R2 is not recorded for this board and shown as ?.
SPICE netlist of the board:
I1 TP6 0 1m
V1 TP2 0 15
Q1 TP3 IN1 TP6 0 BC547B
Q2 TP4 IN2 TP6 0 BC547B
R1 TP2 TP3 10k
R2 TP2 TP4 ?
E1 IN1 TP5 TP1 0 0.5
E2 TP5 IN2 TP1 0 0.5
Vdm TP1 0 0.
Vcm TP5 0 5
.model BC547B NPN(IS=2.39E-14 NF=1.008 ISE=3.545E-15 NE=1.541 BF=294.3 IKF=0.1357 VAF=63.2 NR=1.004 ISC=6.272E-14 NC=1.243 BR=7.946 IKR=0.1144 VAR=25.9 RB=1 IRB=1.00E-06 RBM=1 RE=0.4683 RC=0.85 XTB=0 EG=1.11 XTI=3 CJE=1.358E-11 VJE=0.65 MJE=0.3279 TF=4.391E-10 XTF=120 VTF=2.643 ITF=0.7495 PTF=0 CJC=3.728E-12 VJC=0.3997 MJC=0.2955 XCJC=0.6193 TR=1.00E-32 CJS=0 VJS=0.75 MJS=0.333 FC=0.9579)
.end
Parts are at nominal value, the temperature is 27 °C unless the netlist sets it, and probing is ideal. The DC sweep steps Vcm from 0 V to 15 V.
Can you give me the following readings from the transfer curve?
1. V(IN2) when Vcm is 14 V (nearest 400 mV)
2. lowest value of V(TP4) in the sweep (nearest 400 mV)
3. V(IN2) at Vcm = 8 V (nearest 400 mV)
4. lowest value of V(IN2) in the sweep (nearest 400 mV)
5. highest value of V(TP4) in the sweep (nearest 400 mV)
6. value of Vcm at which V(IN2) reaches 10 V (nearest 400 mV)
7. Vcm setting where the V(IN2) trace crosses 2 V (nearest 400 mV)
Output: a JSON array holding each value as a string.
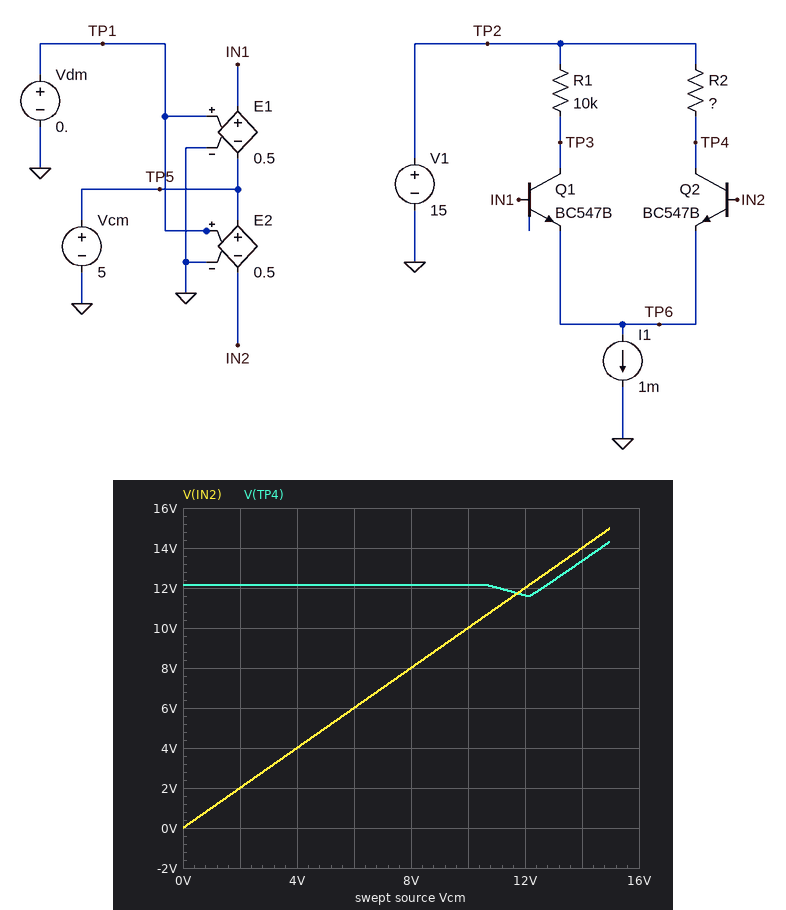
["14.0 V", "11.6 V", "8.0 V", "0 V", "14.4 V", "10.0 V", "2.0 V"]
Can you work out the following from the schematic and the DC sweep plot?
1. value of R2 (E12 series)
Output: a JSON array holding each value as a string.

["5.6 kΩ"]
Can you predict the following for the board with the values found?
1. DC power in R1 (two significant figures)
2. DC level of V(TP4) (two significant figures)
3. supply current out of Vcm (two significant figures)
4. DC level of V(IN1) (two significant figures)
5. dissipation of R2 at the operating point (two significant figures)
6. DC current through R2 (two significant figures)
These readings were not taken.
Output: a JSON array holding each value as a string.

["2.4 mW", "12 V", "3.2 µA", "5.0 V", "1.4 mW", "510 µA"]
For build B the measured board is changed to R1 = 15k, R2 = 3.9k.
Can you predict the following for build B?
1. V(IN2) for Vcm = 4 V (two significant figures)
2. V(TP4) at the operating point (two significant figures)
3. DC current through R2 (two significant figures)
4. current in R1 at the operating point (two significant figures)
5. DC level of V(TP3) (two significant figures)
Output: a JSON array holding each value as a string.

["4.0 V", "13 V", "520 µA", "480 µA", "7.8 V"]
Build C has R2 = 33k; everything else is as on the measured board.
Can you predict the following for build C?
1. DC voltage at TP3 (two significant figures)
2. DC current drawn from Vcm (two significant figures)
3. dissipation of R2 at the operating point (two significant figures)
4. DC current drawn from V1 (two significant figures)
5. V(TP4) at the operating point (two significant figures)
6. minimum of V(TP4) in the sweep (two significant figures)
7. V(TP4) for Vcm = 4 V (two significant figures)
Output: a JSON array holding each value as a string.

["8.6 V", "43 µA", "3.4 mW", "960 µA", "4.4 V", "-230 mV", "3.4 V"]
